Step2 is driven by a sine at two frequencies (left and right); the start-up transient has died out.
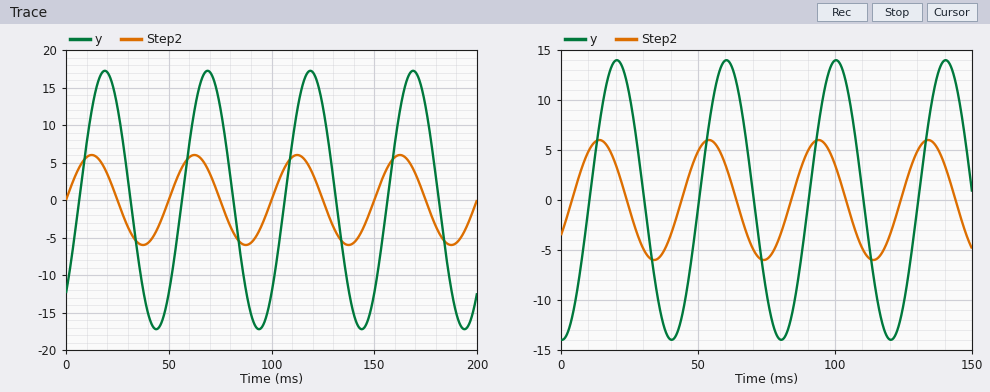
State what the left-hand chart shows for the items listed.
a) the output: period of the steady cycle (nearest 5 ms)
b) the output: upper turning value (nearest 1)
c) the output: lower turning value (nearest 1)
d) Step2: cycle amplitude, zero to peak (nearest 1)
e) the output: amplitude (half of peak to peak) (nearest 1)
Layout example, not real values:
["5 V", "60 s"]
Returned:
["50 ms", "17", "-17", "6", "17"]
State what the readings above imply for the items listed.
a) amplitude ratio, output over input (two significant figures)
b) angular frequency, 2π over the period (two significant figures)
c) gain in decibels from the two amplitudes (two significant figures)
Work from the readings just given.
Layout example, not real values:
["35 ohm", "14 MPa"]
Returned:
["2.8", "0.13 rad/ms", "9.0 dB"]
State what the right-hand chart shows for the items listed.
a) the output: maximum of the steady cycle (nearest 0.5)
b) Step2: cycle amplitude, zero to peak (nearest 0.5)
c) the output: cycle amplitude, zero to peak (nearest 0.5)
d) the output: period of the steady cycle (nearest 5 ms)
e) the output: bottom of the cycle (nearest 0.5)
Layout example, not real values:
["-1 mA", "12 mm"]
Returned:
["14.0", "6.0", "14.0", "40 ms", "-14.0"]
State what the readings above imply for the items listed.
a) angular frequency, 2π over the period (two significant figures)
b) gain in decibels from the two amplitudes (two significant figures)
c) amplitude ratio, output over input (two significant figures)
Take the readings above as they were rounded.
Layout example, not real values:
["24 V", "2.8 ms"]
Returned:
["0.16 rad/ms", "7.4 dB", "2.3"]
